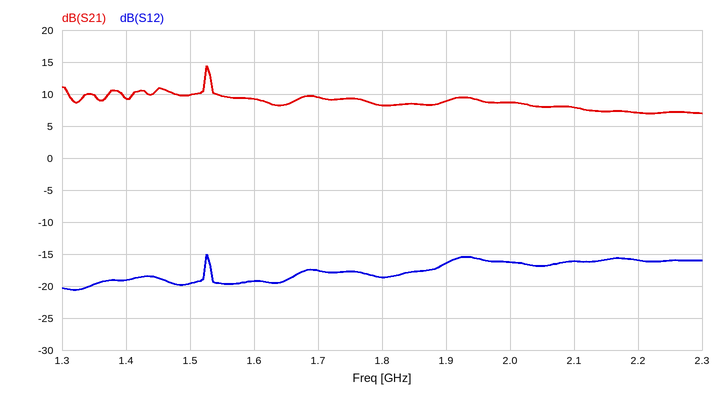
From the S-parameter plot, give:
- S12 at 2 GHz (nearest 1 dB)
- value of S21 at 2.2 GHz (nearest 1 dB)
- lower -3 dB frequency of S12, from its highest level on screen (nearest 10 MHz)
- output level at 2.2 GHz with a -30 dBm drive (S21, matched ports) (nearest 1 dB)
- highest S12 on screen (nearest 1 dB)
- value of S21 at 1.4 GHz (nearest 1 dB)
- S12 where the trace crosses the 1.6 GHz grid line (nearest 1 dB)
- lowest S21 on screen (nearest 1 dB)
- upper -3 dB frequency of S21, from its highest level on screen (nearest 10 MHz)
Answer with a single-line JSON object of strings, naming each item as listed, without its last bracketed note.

{"S12 at 2 GHz": "-16 dB", "value of S21 at 2.2 GHz": "7 dB", "lower -3 dB frequency of S12, from its highest level on screen": "1.52 GHz", "output level at 2.2 GHz with a -30 dBm drive (S21, matched ports)": "-23 dBm", "highest S12 on screen": "-15 dB", "value of S21 at 1.4 GHz": "9 dB", "S12 where the trace crosses the 1.6 GHz grid line": "-19 dB", "lowest S21 on screen": "7 dB", "upper -3 dB frequency of S21, from its highest level on screen": "1.53 GHz"}
